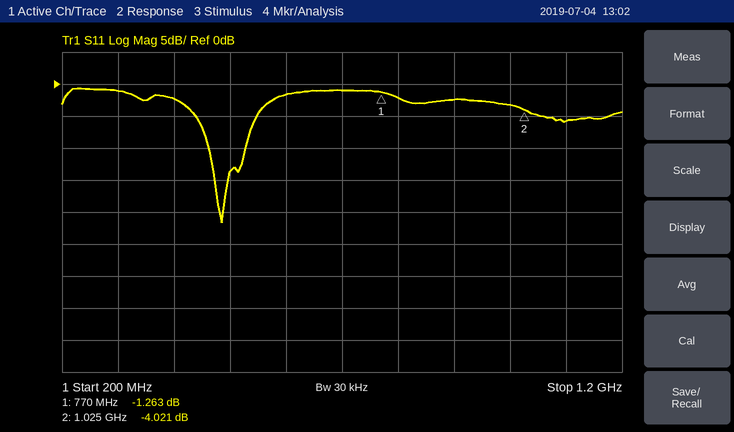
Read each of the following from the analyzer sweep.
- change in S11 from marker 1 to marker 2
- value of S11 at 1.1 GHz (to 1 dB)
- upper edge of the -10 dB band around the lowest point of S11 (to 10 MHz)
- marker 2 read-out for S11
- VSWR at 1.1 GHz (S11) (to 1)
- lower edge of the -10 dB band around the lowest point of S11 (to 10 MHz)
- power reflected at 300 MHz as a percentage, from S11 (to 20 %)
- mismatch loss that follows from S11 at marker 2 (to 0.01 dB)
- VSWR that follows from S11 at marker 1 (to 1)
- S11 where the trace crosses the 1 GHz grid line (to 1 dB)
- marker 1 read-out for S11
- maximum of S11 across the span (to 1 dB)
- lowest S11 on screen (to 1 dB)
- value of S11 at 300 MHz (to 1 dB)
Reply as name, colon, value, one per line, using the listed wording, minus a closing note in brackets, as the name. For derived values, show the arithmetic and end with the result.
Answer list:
change in S11 from marker 1 to marker 2: -4.021 − (-1.263) = -2.758 dB
value of S11 at 1.1 GHz: -6 dB
upper edge of the -10 dB band around the lowest point of S11: 530 MHz
marker 2 read-out for S11: -4.021 dB
VSWR at 1.1 GHz (S11): |Γ| = 10^(-6/20) = 0.5012; VSWR = (1 + 0.5012)/(1 − 0.5012) ≈ 3
lower edge of the -10 dB band around the lowest point of S11: 460 MHz
power reflected at 300 MHz as a percentage, from S11: 10^(-1/10) ≈ 79.4 %, so 80 % to the nearest 20 %
mismatch loss that follows from S11 at marker 2: −10 log10(1 − 10^(-4.021/10)) ≈ 2.19 dB
VSWR that follows from S11 at marker 1: (1 + 0.8647)/(1 − 0.8647) ≈ 14
S11 where the trace crosses the 1 GHz grid line: -3 dB
marker 1 read-out for S11: -1.263 dB
maximum of S11 across the span: -1 dB
lowest S11 on screen: -22 dB
value of S11 at 300 MHz: -1 dB
